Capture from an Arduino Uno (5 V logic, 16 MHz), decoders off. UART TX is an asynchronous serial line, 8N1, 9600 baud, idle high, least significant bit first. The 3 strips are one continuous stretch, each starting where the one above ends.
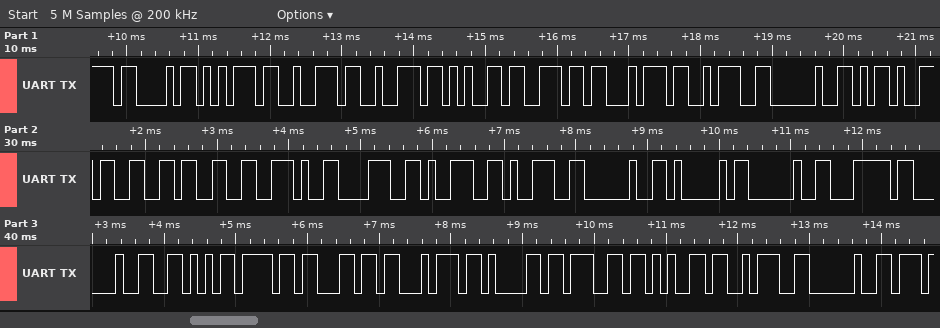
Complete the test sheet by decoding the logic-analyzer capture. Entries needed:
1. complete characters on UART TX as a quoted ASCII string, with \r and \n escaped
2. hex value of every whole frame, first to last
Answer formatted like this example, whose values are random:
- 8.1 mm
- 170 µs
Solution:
- "Current: -33.899 A | Voltage: "
- 43 75 72 72 65 6E 74 3A 20 2D 33 33 2E 38 39 39 20 41 20 7C 20 56 6F 6C 74 61 67 65 3A 20
